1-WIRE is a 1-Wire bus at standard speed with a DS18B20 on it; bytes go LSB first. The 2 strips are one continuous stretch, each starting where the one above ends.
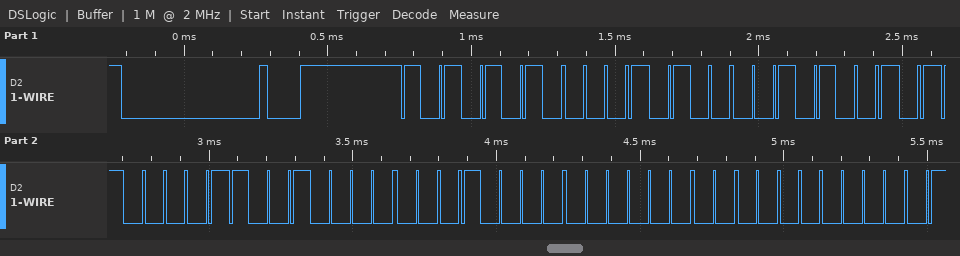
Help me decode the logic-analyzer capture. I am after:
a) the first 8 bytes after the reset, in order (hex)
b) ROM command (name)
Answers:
55 28 94 86 09 08 00 00
Match ROM
